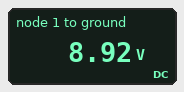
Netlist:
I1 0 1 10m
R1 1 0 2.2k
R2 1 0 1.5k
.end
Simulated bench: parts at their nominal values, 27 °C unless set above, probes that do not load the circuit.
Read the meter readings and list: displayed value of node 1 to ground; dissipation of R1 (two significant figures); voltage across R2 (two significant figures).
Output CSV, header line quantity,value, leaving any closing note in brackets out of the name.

quantity,value
displayed value of node 1 to ground,8.92 V
dissipation of R1,36 mW
voltage across R2,8.9 V
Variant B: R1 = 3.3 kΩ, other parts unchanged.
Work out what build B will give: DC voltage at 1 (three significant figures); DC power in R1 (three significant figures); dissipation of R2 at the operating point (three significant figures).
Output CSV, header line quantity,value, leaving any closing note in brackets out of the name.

quantity,value
DC voltage at 1,10.3 V
DC power in R1,32.2 mW
dissipation of R2 at the operating point,70.9 mW
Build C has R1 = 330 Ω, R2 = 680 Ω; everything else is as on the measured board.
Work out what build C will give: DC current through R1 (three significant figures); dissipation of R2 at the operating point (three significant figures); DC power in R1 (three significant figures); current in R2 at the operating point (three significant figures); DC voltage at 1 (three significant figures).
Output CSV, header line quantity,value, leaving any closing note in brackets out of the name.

quantity,value
DC current through R1,6.73 mA
dissipation of R2 at the operating point,7.26 mW
DC power in R1,15.0 mW
current in R2 at the operating point,3.27 mA
DC voltage at 1,2.22 V
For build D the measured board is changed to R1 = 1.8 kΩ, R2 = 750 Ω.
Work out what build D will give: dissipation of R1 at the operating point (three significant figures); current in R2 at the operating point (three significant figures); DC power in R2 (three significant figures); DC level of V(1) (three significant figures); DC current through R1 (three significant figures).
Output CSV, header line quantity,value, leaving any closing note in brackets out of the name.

quantity,value
dissipation of R1 at the operating point,15.6 mW
current in R2 at the operating point,7.06 mA
DC power in R2,37.4 mW
DC level of V(1),5.29 V
DC current through R1,2.94 mA
